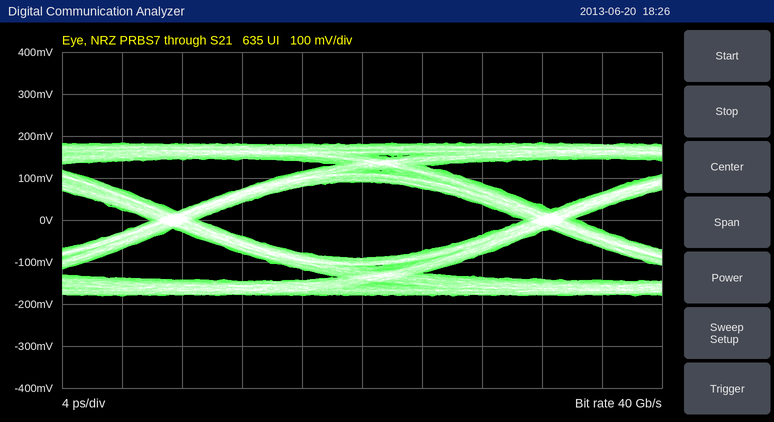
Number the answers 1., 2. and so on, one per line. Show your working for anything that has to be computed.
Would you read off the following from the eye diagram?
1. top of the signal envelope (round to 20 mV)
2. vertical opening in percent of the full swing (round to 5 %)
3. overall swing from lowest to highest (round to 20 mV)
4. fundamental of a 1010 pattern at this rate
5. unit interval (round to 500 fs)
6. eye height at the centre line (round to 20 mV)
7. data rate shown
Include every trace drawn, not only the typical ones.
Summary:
1. 180 mV
2. 180 mV / 360 mV ≈ 50 %
3. 360 mV
4. 20 GHz
5. 25.0 ps
6. 180 mV
7. 40 Gb/s
